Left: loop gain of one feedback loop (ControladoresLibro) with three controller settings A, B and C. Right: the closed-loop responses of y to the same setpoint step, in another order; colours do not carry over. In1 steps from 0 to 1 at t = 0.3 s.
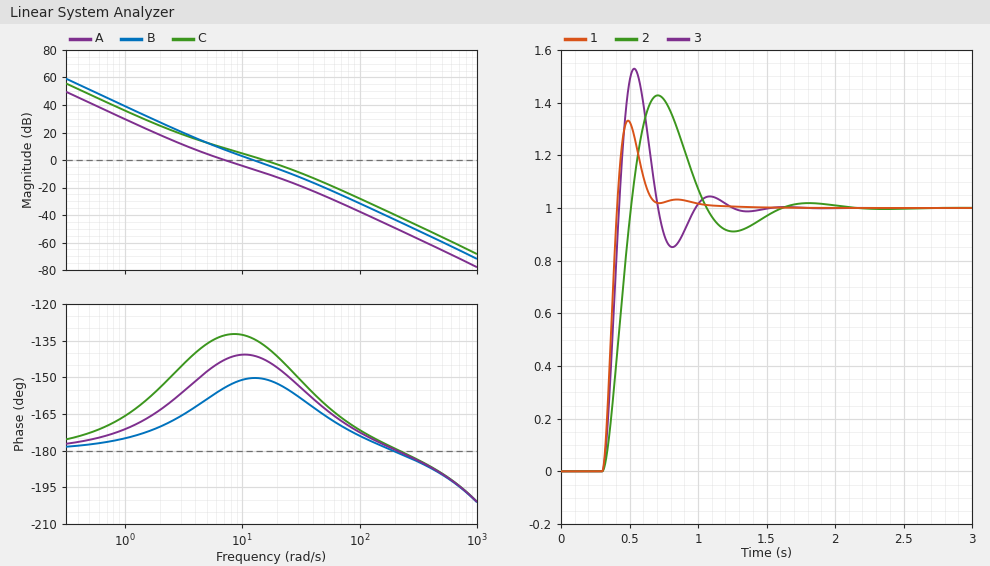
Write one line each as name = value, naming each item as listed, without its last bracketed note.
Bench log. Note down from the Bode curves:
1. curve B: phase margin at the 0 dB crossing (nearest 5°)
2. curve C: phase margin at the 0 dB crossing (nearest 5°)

curve B: phase margin at the 0 dB crossing = 30°
curve C: phase margin at the 0 dB crossing = 45°
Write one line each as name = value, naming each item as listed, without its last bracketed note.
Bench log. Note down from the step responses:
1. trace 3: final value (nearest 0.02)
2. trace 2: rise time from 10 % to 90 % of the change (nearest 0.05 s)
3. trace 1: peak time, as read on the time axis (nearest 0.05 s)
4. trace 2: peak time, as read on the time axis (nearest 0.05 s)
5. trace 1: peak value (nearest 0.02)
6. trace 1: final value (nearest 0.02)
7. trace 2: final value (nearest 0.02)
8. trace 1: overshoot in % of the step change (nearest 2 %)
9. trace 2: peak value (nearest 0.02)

trace 3: final value = 1.00
trace 2: rise time from 10 % to 90 % of the change = 0.15 s
trace 1: peak time, as read on the time axis = 0.50 s
trace 2: peak time, as read on the time axis = 0.70 s
trace 1: peak value = 1.34
trace 1: final value = 1.00
trace 2: final value = 1.00
trace 1: overshoot in % of the step change = 34 %
trace 2: peak value = 1.42
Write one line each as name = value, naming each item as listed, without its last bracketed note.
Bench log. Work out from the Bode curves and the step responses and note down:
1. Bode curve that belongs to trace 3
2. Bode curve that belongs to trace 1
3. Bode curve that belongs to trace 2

Bode curve that belongs to trace 3 = B
Bode curve that belongs to trace 1 = C
Bode curve that belongs to trace 2 = A
